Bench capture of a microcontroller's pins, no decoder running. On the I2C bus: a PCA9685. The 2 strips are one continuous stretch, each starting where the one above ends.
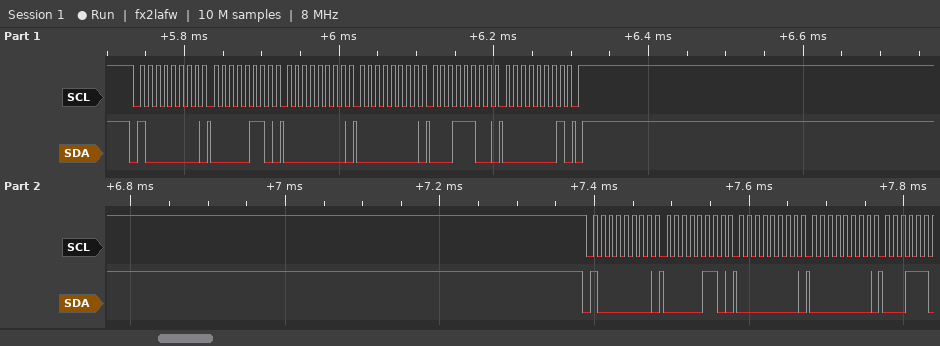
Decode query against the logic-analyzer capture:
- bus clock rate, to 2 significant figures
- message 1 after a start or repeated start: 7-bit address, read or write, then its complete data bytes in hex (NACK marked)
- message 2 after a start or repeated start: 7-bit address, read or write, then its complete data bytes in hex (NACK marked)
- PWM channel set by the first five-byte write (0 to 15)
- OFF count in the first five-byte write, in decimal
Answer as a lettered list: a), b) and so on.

a) 100 kHz
b) 0x40 write: 06 00 00 1C 01
c) 0x40 write: 06 00 00
d) 0
e) 284
